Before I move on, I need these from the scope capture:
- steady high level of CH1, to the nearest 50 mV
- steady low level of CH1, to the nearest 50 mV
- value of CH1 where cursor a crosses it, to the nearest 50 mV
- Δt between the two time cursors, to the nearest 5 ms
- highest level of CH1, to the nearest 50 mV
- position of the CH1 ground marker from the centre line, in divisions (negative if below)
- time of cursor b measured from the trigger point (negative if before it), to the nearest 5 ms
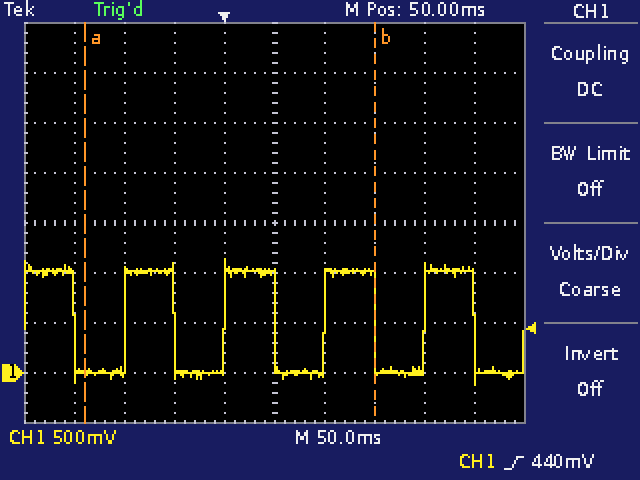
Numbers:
1.00 V
0 mV
0 mV
290 ms
1.15 V
-3.0 div
+150 ms
